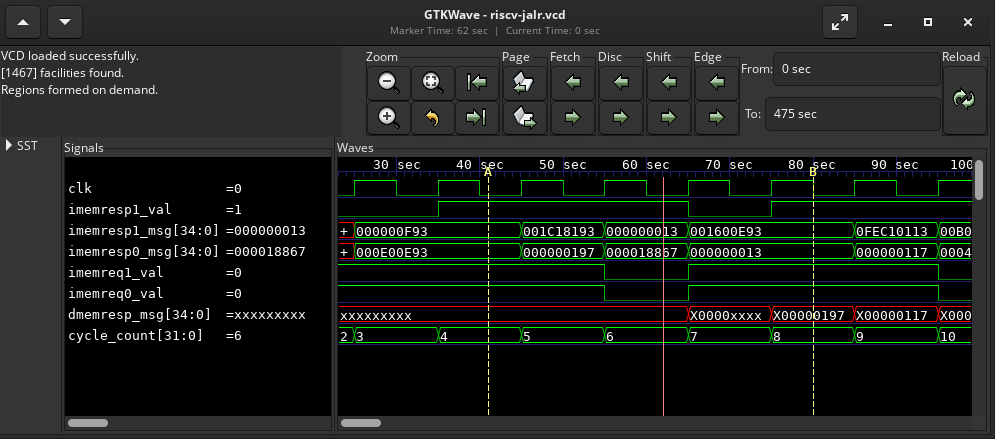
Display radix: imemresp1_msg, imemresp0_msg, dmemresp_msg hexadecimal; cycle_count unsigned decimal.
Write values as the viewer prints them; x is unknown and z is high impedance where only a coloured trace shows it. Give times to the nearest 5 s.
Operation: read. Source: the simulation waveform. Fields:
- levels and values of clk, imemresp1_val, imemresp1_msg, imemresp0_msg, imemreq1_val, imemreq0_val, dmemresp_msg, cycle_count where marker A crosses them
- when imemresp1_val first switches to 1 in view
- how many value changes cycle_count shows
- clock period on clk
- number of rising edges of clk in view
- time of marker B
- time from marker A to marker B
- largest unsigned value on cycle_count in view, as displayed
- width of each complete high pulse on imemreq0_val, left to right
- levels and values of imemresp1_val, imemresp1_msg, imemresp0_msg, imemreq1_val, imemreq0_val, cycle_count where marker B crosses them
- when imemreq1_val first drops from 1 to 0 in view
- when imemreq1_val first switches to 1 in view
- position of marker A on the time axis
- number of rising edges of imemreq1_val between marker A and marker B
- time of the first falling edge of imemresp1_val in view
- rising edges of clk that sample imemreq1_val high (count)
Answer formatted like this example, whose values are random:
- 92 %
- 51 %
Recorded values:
- clk=0, imemresp1_val=1, imemresp1_msg=000000F93, imemresp0_msg=000E00E93, imemreq1_val=1, imemreq0_val=1, dmemresp_msg=xxxxxxxxx, cycle_count=4
- 35 s
- 8
- 10 s
- 8
- 80 s
- 40 s
- 10
- 30 s
- imemresp1_val=1, imemresp1_msg=001600E93, imemresp0_msg=000000013, imemreq1_val=1, imemreq0_val=1, cycle_count=8
- 55 s
- 65 s
- 40 s
- 1
- 65 s
- 7
